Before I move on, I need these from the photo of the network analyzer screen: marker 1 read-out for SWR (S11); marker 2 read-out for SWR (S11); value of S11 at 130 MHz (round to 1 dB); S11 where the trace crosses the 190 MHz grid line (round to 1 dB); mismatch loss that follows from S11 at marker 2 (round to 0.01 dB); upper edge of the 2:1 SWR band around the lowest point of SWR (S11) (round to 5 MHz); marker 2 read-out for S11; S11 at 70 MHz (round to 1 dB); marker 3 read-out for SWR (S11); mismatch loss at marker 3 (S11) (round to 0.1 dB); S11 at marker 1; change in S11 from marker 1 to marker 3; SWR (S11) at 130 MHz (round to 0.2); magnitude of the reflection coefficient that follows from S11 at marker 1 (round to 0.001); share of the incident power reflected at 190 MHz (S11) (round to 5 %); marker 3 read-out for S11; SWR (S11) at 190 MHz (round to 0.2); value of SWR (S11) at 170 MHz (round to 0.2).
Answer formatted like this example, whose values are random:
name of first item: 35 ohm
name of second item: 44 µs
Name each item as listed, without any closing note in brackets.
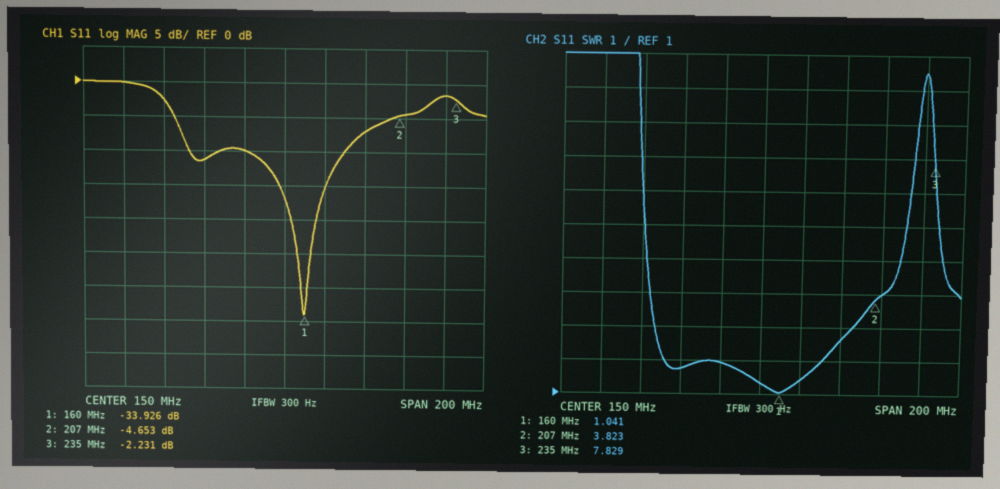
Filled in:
marker 1 read-out for SWR: 1.041
marker 2 read-out for SWR: 3.823
value of S11 at 130 MHz: -10 dB
S11 where the trace crosses the 190 MHz grid line: -7 dB
mismatch loss that follows from S11 at marker 2: 1.82 dB
upper edge of the 2:1 SWR band around the lowest point of SWR (S11): 180 MHz
marker 2 read-out for S11: -4.653 dB
S11 at 70 MHz: 0 dB
marker 3 read-out for SWR: 7.829
mismatch loss at marker 3 (S11): 4.0 dB
S11 at marker 1: -33.926 dB
change in S11 from marker 1 to marker 3: 31.695 dB
SWR (S11) at 130 MHz: 2.0
magnitude of the reflection coefficient that follows from S11 at marker 1: 0.020
share of the incident power reflected at 190 MHz (S11): 20 %
marker 3 read-out for S11: -2.231 dB
SWR (S11) at 190 MHz: 2.6
value of SWR (S11) at 170 MHz: 1.4
